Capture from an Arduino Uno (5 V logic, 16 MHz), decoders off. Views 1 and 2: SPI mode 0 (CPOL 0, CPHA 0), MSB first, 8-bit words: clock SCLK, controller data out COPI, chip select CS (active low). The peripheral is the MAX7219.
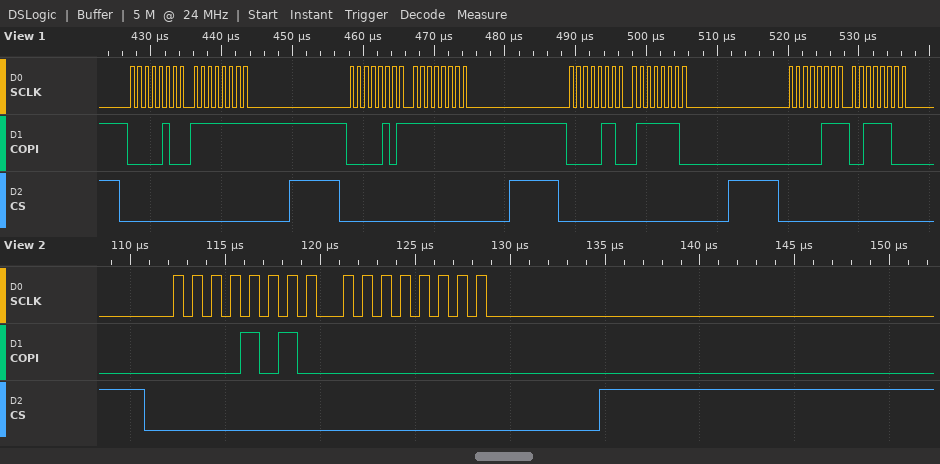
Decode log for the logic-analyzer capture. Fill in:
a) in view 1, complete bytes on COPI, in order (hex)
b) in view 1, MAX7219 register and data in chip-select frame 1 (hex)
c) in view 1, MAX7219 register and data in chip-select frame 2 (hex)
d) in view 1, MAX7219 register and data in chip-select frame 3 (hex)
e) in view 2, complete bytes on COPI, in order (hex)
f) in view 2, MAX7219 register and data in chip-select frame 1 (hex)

04 FF 05 FF 06 7E 07 3C
register 0x4, data 0xFF
register 0x5, data 0xFF
register 0x6, data 0x7E
0x0A 0x00
register 0xA, data 0x00
